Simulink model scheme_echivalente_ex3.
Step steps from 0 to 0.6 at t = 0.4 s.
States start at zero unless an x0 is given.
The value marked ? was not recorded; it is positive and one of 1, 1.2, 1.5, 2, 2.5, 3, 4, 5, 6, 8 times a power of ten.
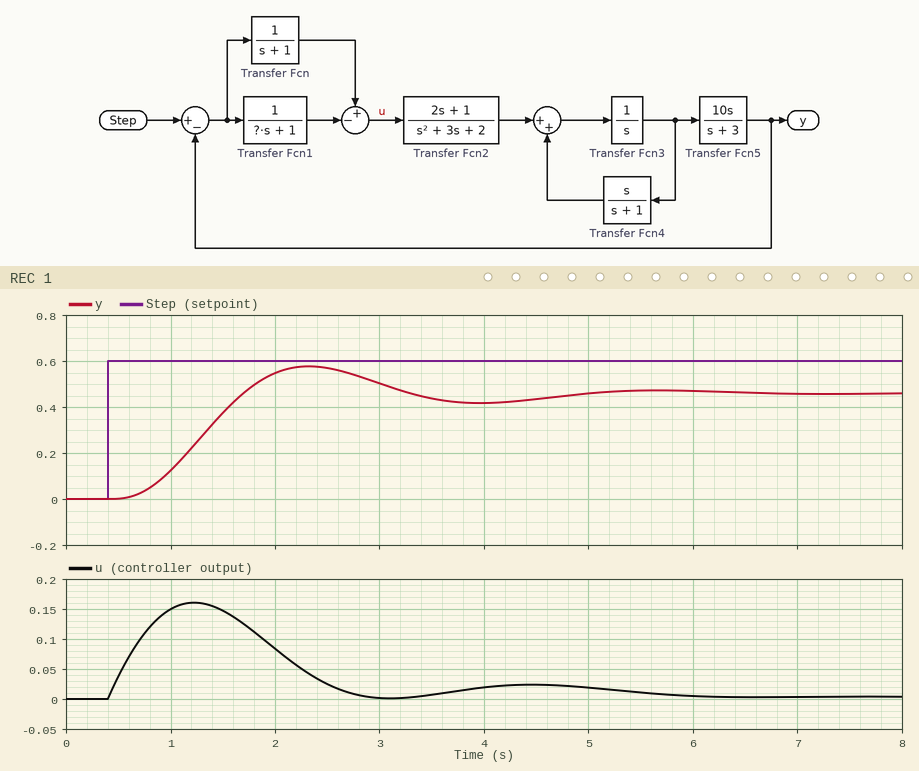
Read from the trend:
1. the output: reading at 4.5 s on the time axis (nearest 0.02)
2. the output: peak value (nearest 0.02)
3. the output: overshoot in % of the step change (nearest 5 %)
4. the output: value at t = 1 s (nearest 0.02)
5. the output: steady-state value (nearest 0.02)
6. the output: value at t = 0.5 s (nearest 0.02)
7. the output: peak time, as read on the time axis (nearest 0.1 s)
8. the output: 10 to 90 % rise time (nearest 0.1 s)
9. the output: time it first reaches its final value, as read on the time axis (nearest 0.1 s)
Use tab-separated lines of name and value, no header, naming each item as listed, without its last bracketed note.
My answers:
the output: reading at 4.5 s on the time axis	0.44
the output: peak value	0.58
the output: overshoot in % of the step change	25 %
the output: value at t = 1 s	0.12
the output: steady-state value	0.46
the output: value at t = 0.5 s	0.00
the output: peak time, as read on the time axis	2.3 s
the output: 10 to 90 % rise time	0.8 s
the output: time it first reaches its final value, as read on the time axis	1.7 s
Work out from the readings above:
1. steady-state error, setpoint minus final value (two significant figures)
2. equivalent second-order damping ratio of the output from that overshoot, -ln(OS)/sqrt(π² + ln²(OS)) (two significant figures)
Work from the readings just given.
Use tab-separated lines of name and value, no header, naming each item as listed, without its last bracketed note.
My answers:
steady-state error, setpoint minus final value	0.14
equivalent second-order damping ratio of the output from that overshoot, -ln(OS)/sqrt(π² + ln²(OS))	0.40
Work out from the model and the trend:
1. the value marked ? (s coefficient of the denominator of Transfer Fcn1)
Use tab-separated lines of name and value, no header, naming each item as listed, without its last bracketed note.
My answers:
the value marked ?	3
